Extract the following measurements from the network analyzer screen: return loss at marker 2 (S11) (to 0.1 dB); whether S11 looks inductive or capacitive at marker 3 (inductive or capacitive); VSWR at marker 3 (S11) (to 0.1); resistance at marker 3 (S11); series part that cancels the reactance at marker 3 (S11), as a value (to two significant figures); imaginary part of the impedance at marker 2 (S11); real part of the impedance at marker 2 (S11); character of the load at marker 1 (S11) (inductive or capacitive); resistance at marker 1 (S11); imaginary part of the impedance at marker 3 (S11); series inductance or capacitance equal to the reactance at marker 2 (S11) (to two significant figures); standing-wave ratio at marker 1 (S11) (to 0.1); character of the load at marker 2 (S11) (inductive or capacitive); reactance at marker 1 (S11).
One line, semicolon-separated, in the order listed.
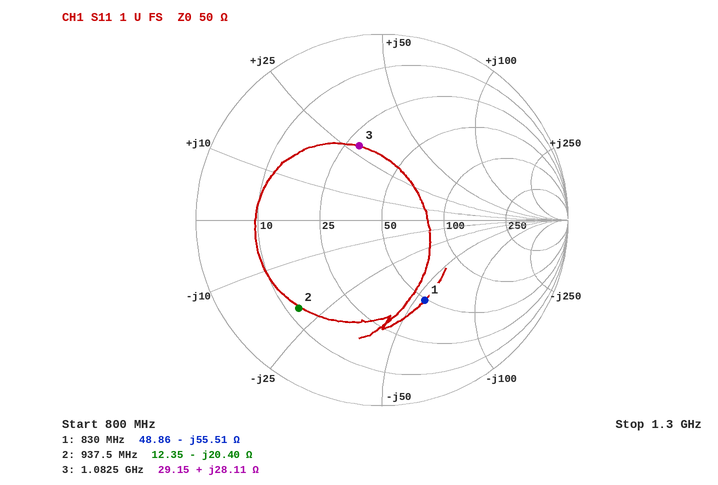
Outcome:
3.7 dB; inductive; 2.4; 29.15 Ω; 5.2 pF; -20.40 Ω; 12.35 Ω; capacitive; 48.86 Ω; +28.11 Ω; 8.3 pF; 2.9; capacitive; -55.51 Ω
